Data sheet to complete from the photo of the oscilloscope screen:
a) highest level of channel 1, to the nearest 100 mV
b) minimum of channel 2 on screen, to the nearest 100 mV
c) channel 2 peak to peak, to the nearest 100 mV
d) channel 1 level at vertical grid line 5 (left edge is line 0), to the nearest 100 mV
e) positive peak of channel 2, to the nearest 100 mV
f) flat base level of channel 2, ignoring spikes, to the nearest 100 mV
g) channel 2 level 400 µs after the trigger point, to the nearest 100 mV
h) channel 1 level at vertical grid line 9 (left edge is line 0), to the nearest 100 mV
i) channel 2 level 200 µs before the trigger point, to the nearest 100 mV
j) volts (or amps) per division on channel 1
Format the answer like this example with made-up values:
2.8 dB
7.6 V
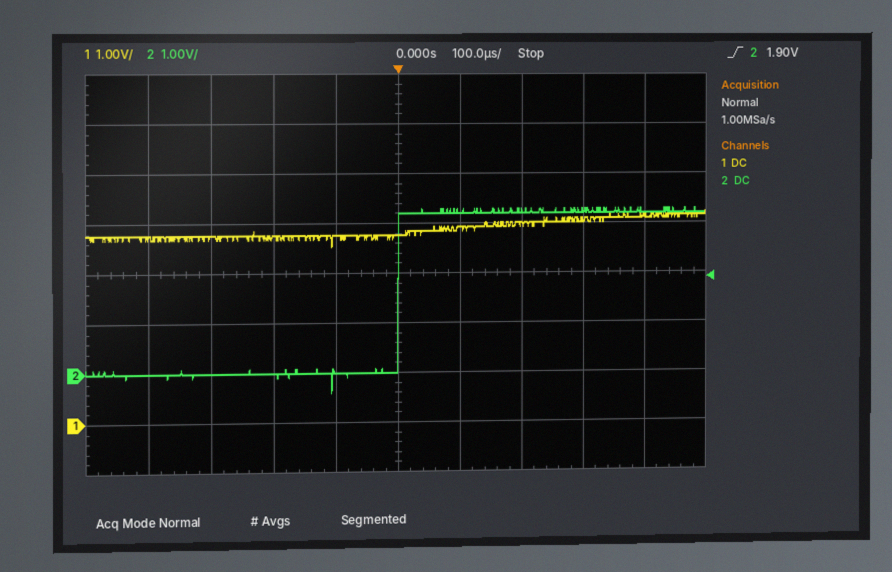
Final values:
4.2 V
-400 mV
3.7 V
3.8 V
3.3 V
0.0 V
3.2 V
4.1 V
0.0 V
1 V
